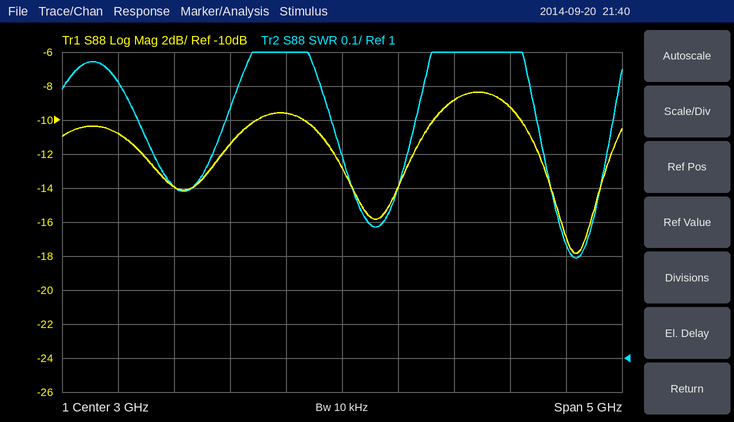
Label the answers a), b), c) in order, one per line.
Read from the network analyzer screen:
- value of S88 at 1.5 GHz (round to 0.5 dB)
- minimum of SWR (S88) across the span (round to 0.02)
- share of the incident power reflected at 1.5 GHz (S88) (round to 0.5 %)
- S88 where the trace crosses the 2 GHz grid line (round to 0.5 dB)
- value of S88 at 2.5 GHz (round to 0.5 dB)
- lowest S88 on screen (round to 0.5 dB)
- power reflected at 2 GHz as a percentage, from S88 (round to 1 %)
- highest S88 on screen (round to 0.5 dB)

a) -14.0 dB
b) 1.30
c) 4.0 %
d) -11.5 dB
e) -9.5 dB
f) -18.0 dB
g) 7 %
h) -8.5 dB
